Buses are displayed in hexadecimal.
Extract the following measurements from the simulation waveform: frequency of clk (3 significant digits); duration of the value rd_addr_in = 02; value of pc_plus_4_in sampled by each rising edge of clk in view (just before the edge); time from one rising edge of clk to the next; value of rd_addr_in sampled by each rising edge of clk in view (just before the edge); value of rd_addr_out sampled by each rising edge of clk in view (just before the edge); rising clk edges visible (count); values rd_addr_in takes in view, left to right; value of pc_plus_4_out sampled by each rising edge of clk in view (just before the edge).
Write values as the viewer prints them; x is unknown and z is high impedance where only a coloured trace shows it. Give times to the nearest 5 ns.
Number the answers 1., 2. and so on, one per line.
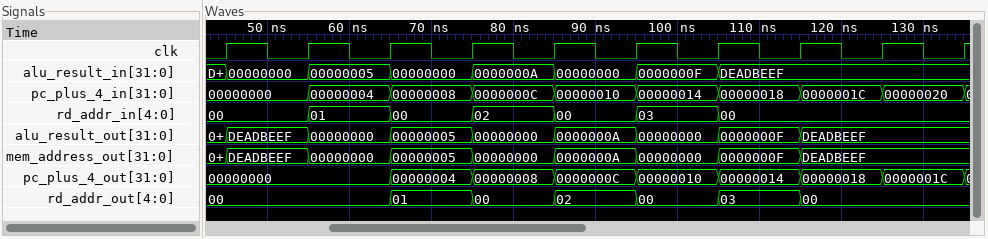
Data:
1. 100 MHz
2. 10 ns
3. 00000000, 00000000, 00000004, 00000008, 0000000C, 00000010, 00000014, 00000018, 0000001C, 00000020
4. 10 ns
5. 00, 00, 01, 00, 02, 00, 03, 00, 00, 00
6. 00, 00, 00, 01, 00, 02, 00, 03, 00, 00
7. 10
8. 00, 01, 00, 02, 00, 03, 00
9. 00000000, 00000000, 00000000, 00000004, 00000008, 0000000C, 00000010, 00000014, 00000018, 0000001C
